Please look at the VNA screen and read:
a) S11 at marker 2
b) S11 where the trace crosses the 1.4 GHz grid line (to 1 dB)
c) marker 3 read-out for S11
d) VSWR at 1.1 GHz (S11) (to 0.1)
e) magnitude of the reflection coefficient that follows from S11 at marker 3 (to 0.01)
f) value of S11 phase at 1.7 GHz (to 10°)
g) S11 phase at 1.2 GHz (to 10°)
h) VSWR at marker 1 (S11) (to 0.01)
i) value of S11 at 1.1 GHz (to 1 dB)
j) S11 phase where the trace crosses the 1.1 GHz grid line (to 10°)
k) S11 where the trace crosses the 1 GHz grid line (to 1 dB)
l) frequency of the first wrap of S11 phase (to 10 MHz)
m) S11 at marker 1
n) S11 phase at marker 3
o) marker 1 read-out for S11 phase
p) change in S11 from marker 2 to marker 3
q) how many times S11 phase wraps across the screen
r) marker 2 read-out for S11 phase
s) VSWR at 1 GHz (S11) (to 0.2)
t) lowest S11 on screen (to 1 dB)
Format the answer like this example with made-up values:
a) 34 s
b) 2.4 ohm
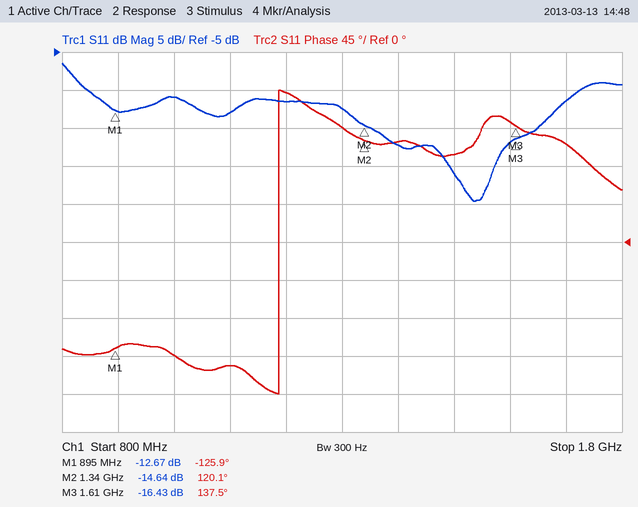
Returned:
a) -14.64 dB
b) -17 dB
c) -16.43 dB
d) 1.6
e) 0.15
f) 120°
g) 180°
h) 1.61
i) -13 dB
j) -150°
k) -11 dB
l) 1.19 GHz
m) -12.67 dB
n) 137.5°
o) -125.9°
p) -1.79 dB
q) 1
r) 120.1°
s) 1.8
t) -25 dB
